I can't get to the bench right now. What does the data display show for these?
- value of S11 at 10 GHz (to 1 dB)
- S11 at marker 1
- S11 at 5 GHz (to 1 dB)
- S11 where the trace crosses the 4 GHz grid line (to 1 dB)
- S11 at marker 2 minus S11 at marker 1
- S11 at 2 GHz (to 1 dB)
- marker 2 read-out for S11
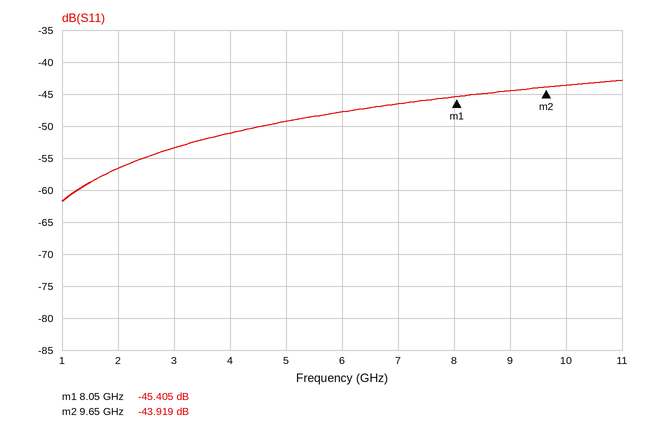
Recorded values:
-44 dB
-45.405 dB
-49 dB
-51 dB
1.486 dB
-57 dB
-43.919 dB
